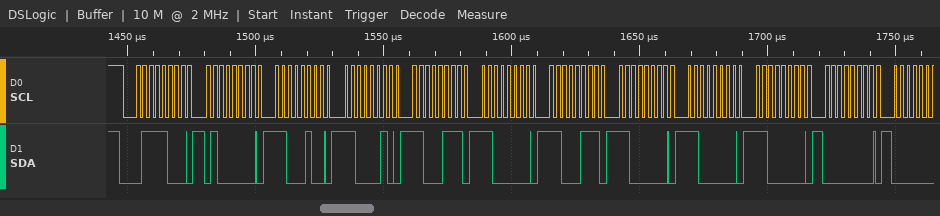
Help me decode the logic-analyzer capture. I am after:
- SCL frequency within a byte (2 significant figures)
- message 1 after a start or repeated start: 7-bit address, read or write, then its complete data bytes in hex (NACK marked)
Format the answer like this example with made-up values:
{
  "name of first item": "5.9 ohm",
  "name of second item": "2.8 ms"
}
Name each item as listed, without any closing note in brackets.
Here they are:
{
  "SCL frequency within a byte": "400 kHz",
  "message 1 after a start or repeated start: 7-bit address, read or write, then its complete data bytes in hex": "0x3C write: 40 C4 C2 C7 C0 C7 C0 C0 C0 00"
}
